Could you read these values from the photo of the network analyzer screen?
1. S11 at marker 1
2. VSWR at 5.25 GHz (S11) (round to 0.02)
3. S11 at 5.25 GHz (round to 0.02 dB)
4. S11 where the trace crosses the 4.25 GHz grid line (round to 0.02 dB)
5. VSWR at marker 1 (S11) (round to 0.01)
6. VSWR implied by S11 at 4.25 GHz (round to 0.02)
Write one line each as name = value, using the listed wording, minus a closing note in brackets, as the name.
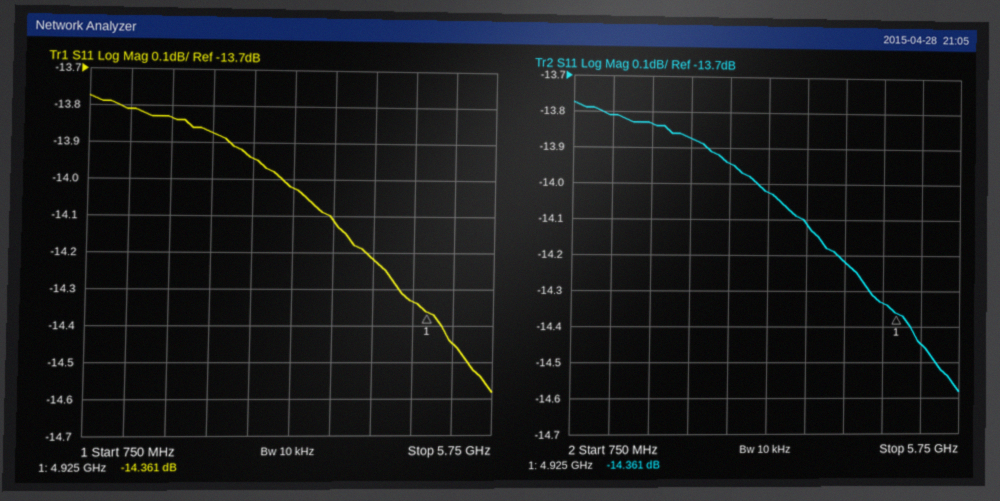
S11 at marker 1 = -14.361 dB
VSWR at 5.25 GHz (S11) = 1.46
S11 at 5.25 GHz = -14.44 dB
S11 where the trace crosses the 4.25 GHz grid line = -14.22 dB
VSWR at marker 1 (S11) = 1.47
VSWR implied by S11 at 4.25 GHz = 1.48
